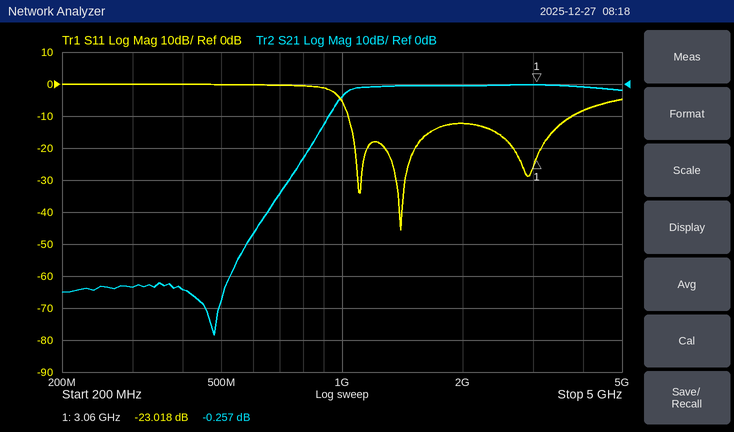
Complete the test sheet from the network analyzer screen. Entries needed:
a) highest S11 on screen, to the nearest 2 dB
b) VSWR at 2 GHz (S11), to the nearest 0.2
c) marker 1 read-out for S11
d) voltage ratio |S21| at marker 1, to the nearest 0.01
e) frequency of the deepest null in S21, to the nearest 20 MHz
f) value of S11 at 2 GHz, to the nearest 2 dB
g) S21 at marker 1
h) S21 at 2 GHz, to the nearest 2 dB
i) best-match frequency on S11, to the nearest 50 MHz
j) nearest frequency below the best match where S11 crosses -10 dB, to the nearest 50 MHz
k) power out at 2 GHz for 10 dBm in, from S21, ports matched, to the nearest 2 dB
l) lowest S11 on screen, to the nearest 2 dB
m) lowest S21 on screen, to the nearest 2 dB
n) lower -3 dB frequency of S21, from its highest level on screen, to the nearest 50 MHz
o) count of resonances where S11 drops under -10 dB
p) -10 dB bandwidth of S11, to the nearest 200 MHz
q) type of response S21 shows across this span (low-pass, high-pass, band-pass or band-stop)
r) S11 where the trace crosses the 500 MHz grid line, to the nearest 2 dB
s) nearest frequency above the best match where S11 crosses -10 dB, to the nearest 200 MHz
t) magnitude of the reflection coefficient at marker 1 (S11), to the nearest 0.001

0 dB
1.6
-23.018 dB
0.97
480 MHz
-12 dB
-0.257 dB
0 dB
1.40 GHz
1.05 GHz
10 dBm
-46 dB
-78 dB
1.00 GHz
3
2.8 GHz
high-pass
0 dB
3.8 GHz
0.071
